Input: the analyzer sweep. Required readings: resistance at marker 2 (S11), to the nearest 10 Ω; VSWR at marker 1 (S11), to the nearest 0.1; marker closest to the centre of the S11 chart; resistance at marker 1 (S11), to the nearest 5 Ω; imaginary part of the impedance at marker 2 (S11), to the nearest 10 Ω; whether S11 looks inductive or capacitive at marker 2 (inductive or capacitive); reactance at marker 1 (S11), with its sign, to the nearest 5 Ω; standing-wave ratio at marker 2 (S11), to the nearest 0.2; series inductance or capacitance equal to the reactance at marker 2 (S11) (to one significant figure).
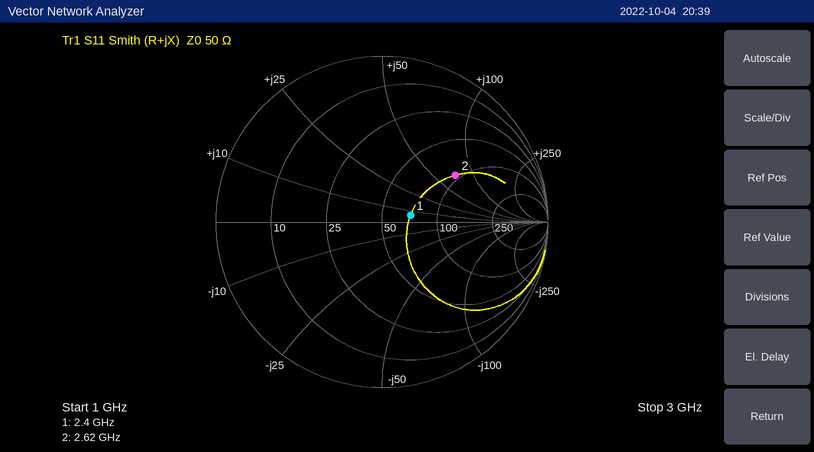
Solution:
90 Ω
1.4
marker 1
70 Ω
+70 Ω
inductive
+5 Ω
3.2
4 nH
